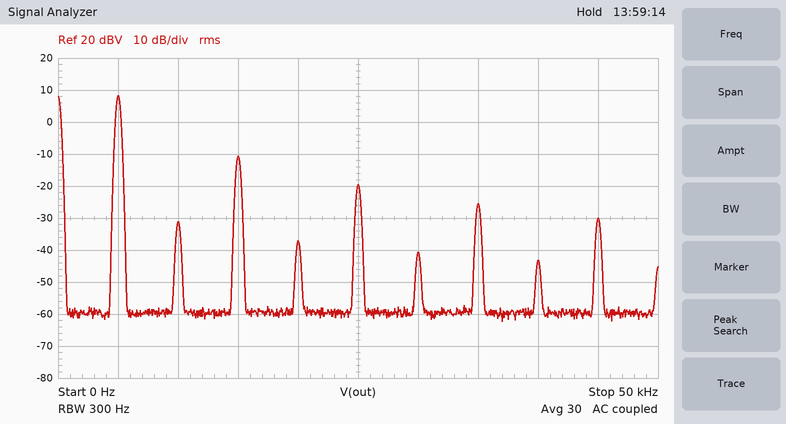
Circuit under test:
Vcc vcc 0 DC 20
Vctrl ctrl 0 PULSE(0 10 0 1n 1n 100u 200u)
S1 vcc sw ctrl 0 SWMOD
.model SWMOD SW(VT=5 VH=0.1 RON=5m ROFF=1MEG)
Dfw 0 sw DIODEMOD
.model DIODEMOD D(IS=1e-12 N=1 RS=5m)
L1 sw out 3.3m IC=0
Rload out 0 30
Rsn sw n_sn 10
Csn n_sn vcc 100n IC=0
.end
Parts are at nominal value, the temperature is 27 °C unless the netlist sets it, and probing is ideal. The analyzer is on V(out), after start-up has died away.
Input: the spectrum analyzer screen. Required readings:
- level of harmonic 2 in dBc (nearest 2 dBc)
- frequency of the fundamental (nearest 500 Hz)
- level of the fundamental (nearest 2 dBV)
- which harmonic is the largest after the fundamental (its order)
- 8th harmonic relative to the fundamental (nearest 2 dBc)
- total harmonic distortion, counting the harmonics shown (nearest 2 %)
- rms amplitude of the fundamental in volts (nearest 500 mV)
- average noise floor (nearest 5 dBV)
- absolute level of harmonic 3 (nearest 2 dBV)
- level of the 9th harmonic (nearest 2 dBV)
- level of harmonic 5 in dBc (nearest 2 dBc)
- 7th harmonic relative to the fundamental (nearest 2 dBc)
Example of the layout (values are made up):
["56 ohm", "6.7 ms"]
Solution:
["-40 dBc", "5.0 kHz", "8 dBV", "3", "-52 dBc", "12 %", "2.5 V", "-60 dBV", "-10 dBV", "-30 dBV", "-28 dBc", "-34 dBc"]
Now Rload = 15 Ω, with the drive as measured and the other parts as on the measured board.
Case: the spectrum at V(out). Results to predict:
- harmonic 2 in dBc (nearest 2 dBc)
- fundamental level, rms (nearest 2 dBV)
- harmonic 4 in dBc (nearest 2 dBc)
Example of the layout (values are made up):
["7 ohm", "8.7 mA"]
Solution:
["-48 dBc", "2 dBV", "-54 dBc"]
